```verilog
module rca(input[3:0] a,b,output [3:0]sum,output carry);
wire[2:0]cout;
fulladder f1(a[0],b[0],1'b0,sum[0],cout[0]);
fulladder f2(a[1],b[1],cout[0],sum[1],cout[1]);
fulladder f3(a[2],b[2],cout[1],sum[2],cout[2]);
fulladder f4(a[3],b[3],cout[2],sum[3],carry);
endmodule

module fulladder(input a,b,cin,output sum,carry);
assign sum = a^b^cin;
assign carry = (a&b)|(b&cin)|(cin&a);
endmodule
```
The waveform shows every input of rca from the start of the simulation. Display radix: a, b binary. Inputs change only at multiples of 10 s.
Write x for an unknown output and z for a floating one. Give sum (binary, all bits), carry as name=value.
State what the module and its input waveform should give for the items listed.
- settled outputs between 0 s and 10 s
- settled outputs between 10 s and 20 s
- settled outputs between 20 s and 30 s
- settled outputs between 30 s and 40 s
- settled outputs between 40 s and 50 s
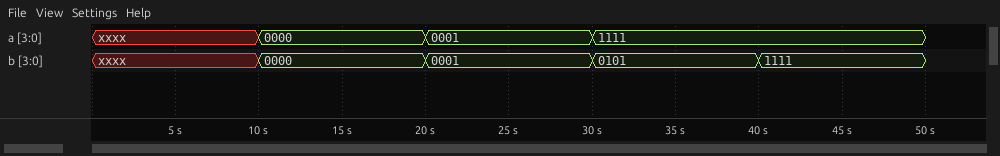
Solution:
sum=x, carry=x
sum=0000, carry=0
sum=0010, carry=0
sum=0100, carry=1
sum=1110, carry=1
